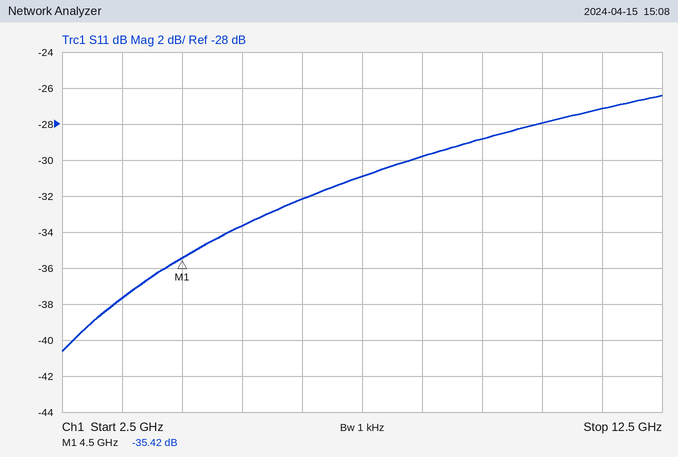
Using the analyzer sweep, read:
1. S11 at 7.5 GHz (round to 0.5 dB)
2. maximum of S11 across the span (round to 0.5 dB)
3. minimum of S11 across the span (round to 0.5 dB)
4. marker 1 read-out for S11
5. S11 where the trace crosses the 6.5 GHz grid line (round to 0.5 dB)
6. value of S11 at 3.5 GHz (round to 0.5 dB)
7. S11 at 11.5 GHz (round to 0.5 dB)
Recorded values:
-31.0 dB
-26.5 dB
-40.5 dB
-35.42 dB
-32.0 dB
-37.5 dB
-27.0 dB
